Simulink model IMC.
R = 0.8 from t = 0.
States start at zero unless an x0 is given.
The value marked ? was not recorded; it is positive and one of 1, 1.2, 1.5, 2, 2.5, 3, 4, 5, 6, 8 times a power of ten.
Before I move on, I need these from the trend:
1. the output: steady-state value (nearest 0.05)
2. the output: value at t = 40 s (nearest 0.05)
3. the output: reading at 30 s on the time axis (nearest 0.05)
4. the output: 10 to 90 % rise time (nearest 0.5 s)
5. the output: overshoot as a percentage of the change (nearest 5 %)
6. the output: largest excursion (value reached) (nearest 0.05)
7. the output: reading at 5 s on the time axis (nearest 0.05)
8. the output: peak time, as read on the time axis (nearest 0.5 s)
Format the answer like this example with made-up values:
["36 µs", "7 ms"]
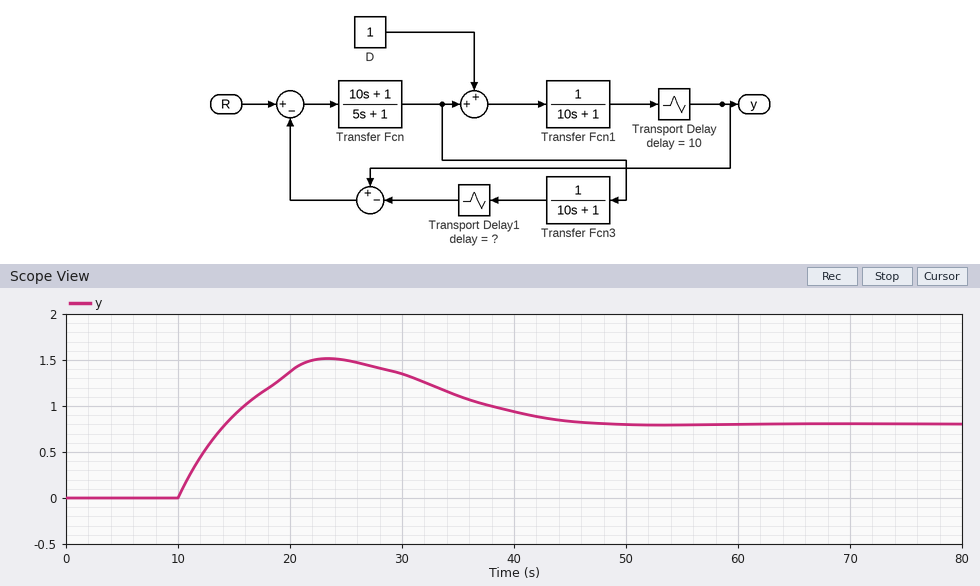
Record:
["0.80", "0.95", "1.35", "3.5 s", "90 %", "1.50", "0.00", "23.5 s"]
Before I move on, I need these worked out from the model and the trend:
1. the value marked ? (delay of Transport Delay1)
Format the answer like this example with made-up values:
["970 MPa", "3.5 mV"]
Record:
["8"]
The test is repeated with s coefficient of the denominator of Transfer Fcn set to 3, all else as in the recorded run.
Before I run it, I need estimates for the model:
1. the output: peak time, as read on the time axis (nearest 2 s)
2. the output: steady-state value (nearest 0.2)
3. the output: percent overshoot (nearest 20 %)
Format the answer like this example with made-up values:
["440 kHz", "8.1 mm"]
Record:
["22 s", "0.8", "100 %"]
